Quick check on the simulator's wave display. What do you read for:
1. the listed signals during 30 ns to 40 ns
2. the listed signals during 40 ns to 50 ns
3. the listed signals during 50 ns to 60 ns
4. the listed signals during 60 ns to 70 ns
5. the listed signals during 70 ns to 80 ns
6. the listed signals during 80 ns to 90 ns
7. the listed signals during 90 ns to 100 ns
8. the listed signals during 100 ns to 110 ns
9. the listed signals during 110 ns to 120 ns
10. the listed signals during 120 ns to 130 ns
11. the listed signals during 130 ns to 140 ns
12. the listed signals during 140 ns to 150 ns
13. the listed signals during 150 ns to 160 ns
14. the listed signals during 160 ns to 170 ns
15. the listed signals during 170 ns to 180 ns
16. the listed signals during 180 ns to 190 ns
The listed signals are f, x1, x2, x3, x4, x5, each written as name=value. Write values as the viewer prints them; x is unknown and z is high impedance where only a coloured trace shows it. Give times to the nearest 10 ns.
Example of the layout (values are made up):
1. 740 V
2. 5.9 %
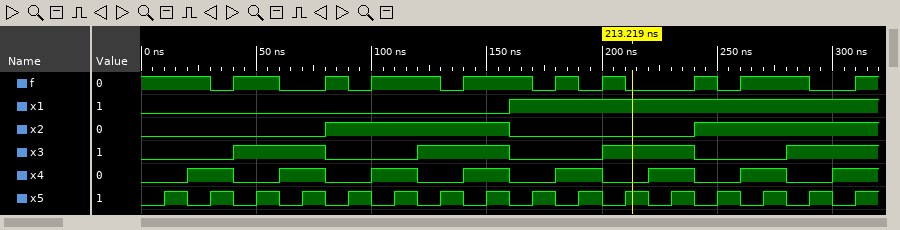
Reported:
1. f=0, x1=0, x2=0, x3=0, x4=1, x5=1
2. f=1, x1=0, x2=0, x3=1, x4=0, x5=0
3. f=1, x1=0, x2=0, x3=1, x4=0, x5=1
4. f=0, x1=0, x2=0, x3=1, x4=1, x5=0
5. f=0, x1=0, x2=0, x3=1, x4=1, x5=1
6. f=1, x1=0, x2=1, x3=0, x4=0, x5=0
7. f=0, x1=0, x2=1, x3=0, x4=0, x5=1
8. f=1, x1=0, x2=1, x3=0, x4=1, x5=0
9. f=1, x1=0, x2=1, x3=0, x4=1, x5=1
10. f=1, x1=0, x2=1, x3=1, x4=0, x5=0
11. f=0, x1=0, x2=1, x3=1, x4=0, x5=1
12. f=1, x1=0, x2=1, x3=1, x4=1, x5=0
13. f=1, x1=0, x2=1, x3=1, x4=1, x5=1
14. f=1, x1=1, x2=0, x3=0, x4=0, x5=0
15. f=0, x1=1, x2=0, x3=0, x4=0, x5=1
16. f=1, x1=1, x2=0, x3=0, x4=1, x5=0
